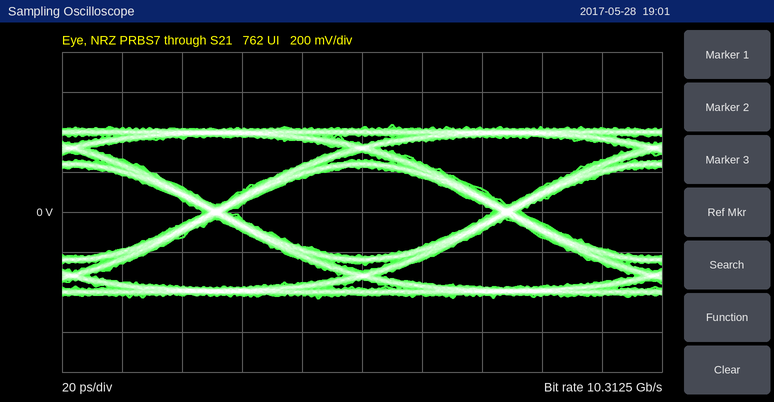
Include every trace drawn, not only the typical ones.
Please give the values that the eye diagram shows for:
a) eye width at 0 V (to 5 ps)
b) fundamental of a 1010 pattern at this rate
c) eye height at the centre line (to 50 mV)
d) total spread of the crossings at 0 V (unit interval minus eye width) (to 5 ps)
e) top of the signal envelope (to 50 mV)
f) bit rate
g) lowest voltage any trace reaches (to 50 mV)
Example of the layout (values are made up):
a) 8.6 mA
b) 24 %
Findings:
a) 90 ps
b) 5.15625 GHz
c) 450 mV
d) 10 ps
e) 450 mV
f) 10.3125 Gb/s
g) -450 mV
